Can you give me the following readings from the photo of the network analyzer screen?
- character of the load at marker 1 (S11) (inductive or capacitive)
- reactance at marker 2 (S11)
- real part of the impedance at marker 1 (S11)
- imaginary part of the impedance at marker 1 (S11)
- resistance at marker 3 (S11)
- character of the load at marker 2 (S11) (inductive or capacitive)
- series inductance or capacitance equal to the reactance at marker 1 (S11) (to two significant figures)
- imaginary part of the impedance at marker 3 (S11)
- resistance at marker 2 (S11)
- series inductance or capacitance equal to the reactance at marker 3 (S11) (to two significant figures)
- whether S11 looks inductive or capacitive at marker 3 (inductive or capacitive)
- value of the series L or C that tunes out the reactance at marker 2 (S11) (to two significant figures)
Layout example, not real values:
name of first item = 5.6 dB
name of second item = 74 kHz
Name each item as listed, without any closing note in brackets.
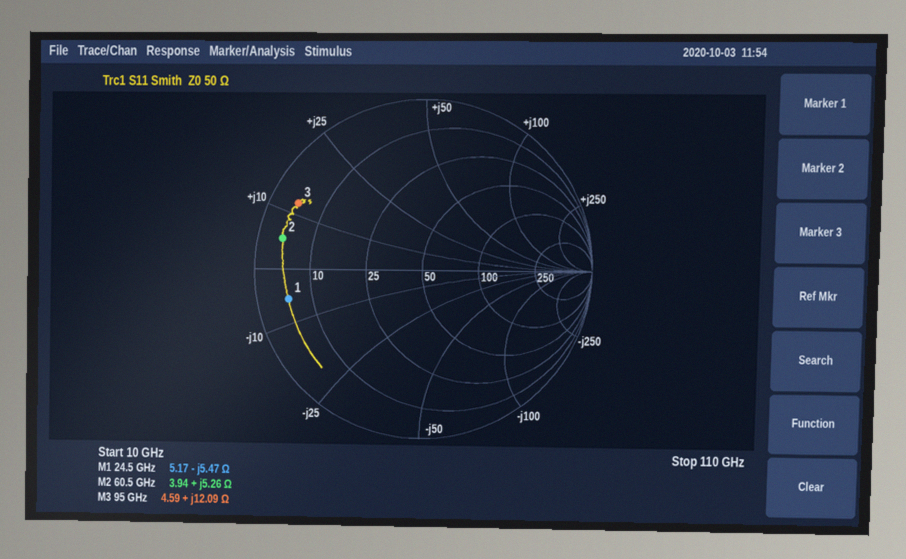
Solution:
character of the load at marker 1 (S11) = capacitive
reactance at marker 2 = +5.26 Ω
real part of the impedance at marker 1 = 5.17 Ω
imaginary part of the impedance at marker 1 = -5.47 Ω
resistance at marker 3 = 4.59 Ω
character of the load at marker 2 (S11) = inductive
series inductance or capacitance equal to the reactance at marker 1 (S11) = 1.2 pF
imaginary part of the impedance at marker 3 = +12.09 Ω
resistance at marker 2 = 3.94 Ω
series inductance or capacitance equal to the reactance at marker 3 (S11) = 20 pH
whether S11 looks inductive or capacitive at marker 3 = inductive
value of the series L or C that tunes out the reactance at marker 2 (S11) = 500 fF
